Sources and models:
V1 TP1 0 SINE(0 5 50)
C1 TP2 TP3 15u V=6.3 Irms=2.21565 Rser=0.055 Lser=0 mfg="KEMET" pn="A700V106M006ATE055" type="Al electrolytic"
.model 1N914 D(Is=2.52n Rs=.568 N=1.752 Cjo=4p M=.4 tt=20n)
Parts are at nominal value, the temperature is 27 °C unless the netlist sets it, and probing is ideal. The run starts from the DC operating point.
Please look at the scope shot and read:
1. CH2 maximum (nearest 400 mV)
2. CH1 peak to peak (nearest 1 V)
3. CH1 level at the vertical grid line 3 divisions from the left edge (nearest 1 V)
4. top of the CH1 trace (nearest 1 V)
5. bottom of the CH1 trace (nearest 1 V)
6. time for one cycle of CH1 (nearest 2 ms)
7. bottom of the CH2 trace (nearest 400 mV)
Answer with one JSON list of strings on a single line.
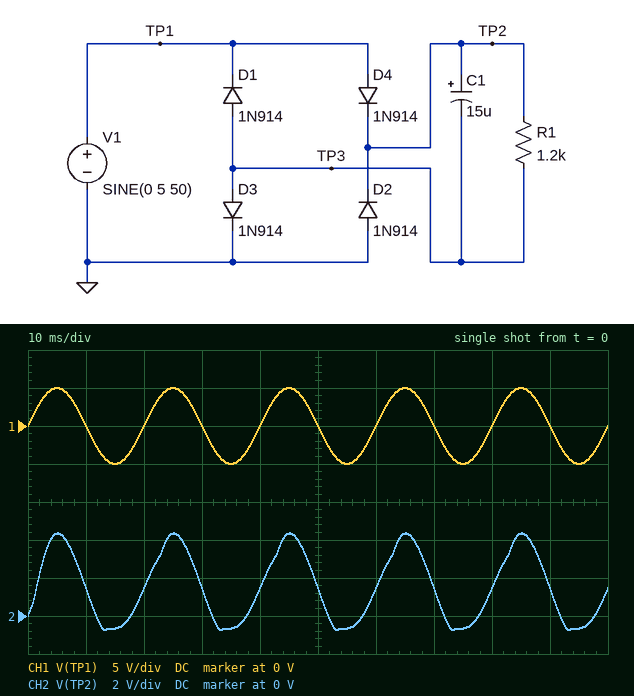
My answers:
["4.4 V", "10 V", "0 V", "5 V", "-5 V", "20 ms", "-800 mV"]
